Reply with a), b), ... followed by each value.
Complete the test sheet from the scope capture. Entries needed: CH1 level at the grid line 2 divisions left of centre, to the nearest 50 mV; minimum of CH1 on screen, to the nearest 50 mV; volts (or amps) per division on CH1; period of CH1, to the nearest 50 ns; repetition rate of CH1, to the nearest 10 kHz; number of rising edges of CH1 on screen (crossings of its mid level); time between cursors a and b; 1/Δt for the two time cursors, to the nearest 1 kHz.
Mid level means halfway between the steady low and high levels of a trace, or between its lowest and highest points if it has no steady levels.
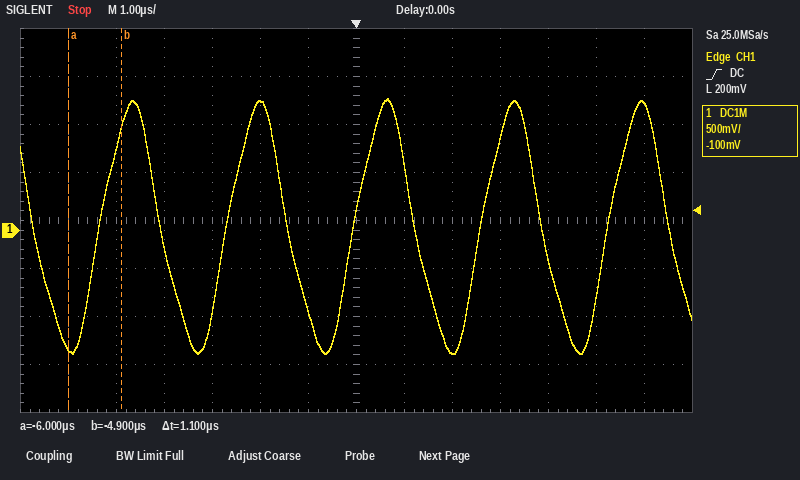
a) 1.35 V
b) -1.30 V
c) 500 mV
d) 2.65 µs
e) 380 kHz
f) 5
g) 1.1 µs
h) 909 kHz
